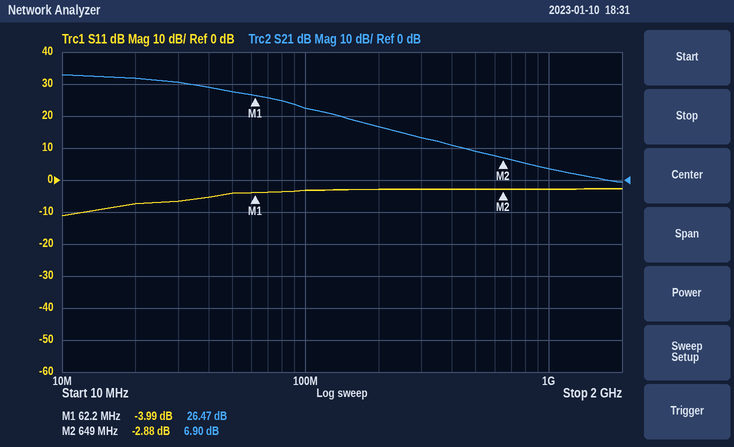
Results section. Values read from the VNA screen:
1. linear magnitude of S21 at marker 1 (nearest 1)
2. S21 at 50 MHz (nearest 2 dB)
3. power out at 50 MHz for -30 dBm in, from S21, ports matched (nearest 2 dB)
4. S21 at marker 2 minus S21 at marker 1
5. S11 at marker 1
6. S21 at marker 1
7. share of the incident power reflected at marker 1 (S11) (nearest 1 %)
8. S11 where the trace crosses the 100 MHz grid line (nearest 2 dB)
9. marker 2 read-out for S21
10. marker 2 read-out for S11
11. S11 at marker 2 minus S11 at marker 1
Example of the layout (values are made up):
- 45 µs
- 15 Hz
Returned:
- 21
- 28 dB
- -2 dBm
- -19.57 dB
- -3.99 dB
- 26.47 dB
- 40 %
- -4 dB
- 6.90 dB
- -2.88 dB
- 1.11 dB
